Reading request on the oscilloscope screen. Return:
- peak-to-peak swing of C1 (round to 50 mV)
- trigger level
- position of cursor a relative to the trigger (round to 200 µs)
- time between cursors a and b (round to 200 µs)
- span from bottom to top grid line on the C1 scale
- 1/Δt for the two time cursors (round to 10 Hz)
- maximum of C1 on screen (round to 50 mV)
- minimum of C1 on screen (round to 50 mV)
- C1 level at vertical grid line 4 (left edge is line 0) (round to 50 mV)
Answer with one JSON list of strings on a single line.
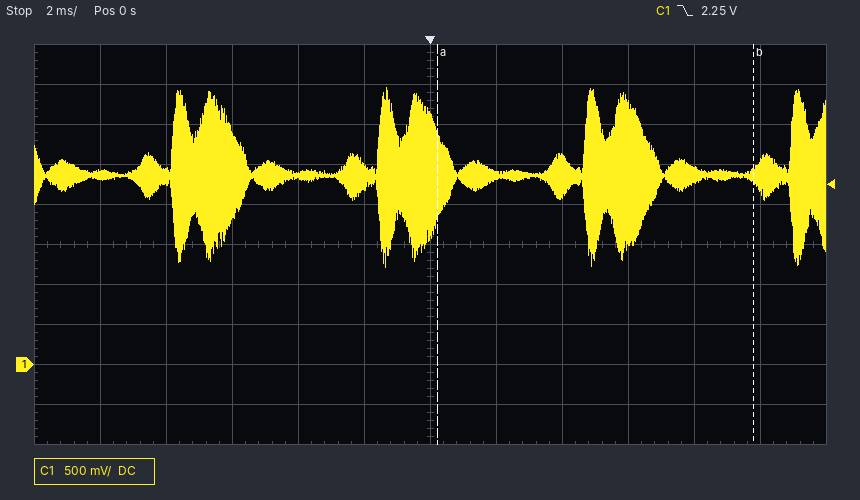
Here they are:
["2.25 V", "2.25 V", "+200 µs", "9.6 ms", "5 V", "100 Hz", "3.45 V", "1.20 V", "2.35 V"]
